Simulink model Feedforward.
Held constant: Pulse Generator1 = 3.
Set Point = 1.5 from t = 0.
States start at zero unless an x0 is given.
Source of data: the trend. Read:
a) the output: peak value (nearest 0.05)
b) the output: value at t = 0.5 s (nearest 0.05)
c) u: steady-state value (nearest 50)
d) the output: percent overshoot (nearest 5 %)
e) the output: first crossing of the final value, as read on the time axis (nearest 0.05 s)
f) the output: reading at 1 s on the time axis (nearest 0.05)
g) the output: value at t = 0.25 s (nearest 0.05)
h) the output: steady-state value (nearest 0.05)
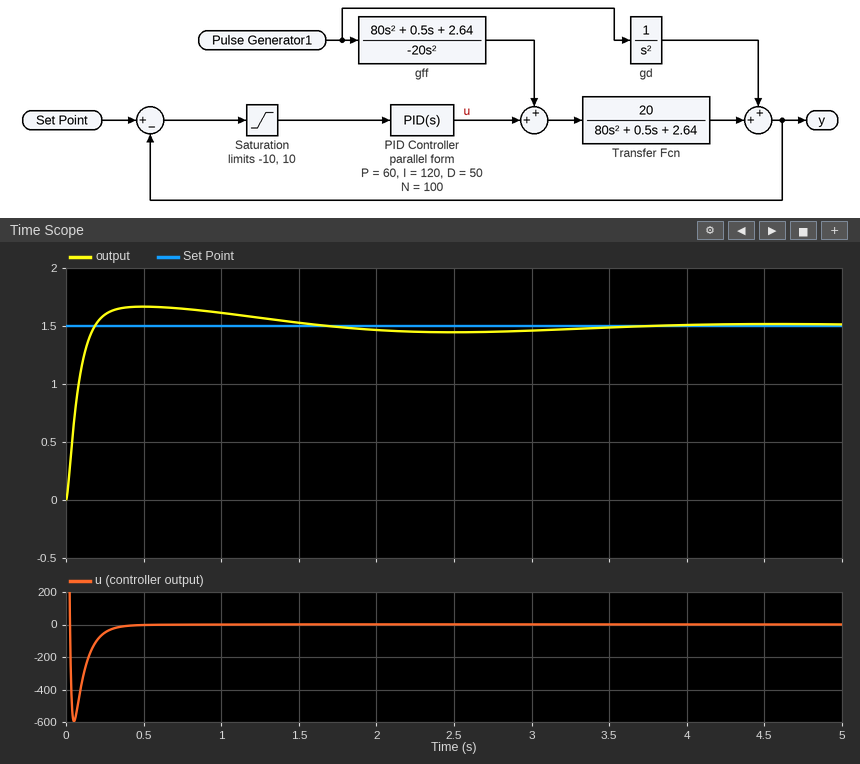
1.65
1.65
0
10 %
0.20 s
1.60
1.60
1.50
